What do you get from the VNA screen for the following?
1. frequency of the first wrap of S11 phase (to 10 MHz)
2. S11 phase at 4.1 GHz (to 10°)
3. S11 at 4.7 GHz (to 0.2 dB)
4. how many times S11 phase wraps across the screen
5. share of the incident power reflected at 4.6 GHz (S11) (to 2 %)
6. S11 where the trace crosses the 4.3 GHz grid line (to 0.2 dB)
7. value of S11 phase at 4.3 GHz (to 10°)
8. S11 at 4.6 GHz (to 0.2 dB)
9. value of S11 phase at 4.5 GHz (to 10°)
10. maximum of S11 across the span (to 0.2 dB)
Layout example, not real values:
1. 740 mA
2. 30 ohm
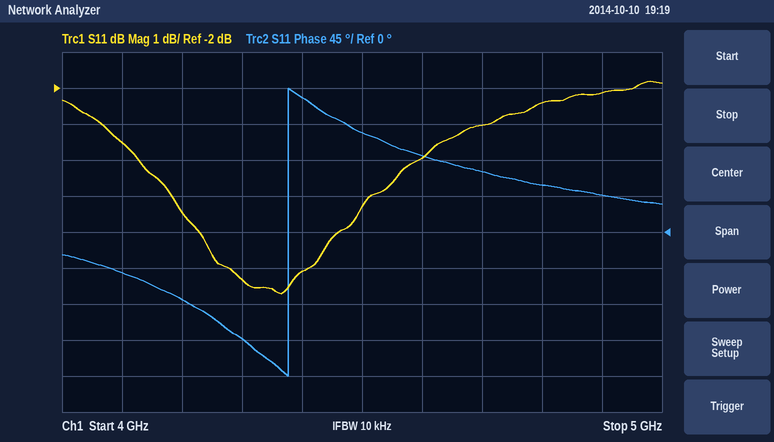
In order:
1. 4.38 GHz
2. -50°
3. -3.0 dB
4. 1
5. 40 %
6. -7.4 dB
7. -130°
8. -4.0 dB
9. 120°
10. -1.8 dB
